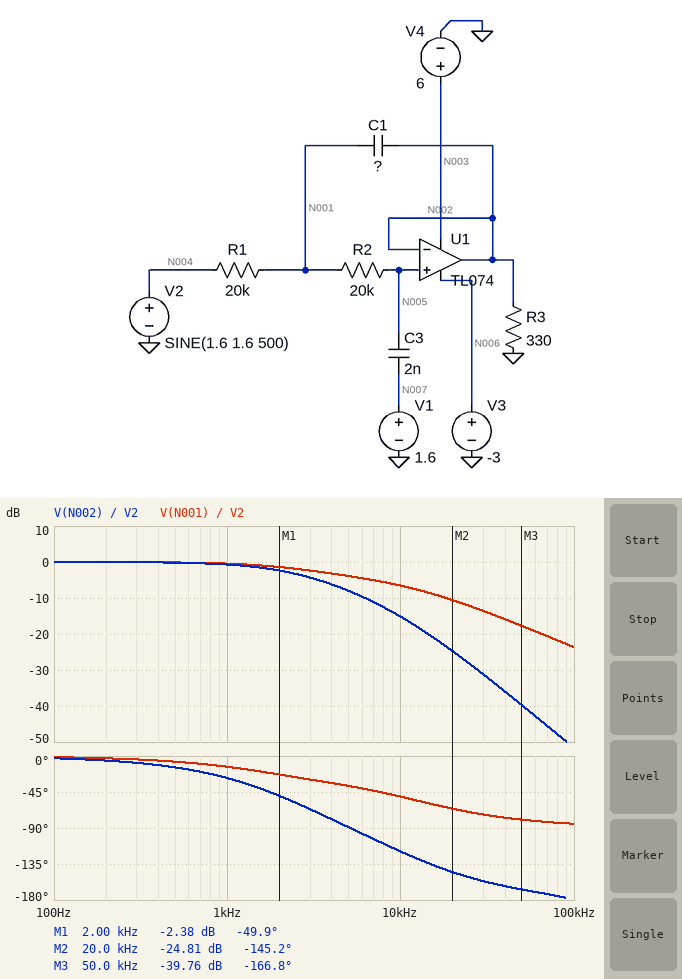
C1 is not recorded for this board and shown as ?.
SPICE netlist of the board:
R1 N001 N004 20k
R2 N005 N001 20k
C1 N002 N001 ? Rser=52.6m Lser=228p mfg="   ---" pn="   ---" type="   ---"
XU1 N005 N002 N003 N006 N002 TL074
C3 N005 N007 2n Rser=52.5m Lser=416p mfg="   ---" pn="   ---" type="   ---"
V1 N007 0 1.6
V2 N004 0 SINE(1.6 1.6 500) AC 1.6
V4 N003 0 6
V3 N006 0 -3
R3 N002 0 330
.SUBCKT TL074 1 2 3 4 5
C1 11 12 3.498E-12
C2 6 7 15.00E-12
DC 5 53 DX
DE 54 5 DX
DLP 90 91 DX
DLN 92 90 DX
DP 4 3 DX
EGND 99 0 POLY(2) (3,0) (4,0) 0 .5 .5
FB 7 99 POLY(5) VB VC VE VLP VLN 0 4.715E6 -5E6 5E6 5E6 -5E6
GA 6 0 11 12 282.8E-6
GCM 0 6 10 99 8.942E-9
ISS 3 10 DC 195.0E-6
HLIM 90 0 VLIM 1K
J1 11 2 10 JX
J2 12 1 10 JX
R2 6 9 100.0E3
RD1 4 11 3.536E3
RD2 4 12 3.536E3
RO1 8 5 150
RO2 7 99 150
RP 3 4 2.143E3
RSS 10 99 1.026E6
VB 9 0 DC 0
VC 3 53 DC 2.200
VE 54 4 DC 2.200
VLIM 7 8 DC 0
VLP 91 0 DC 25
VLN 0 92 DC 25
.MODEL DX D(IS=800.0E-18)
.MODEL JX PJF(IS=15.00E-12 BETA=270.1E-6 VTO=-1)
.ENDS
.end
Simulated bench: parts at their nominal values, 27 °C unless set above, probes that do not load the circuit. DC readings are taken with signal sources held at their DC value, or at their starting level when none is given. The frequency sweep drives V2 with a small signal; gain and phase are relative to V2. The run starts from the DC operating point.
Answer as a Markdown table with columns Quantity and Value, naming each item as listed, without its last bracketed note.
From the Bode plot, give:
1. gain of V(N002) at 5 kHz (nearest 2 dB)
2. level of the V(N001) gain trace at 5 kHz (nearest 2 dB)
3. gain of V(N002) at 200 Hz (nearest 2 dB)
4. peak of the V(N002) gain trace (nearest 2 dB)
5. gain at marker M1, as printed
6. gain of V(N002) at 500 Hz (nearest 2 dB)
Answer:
| Quantity | Value |
|---|---|
| gain of V(N002) at 5 kHz | -8 dB |
| level of the V(N001) gain trace at 5 kHz | -4 dB |
| gain of V(N002) at 200 Hz | 0 dB |
| peak of the V(N002) gain trace | 0 dB |
| gain at marker M1, as printed | -2.38 dB |
| gain of V(N002) at 500 Hz | 0 dB |
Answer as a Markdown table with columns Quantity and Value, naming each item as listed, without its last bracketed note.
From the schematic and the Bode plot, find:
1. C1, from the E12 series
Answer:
| Quantity | Value |
|---|---|
| C1, from the E12 series | 1.2 nF |
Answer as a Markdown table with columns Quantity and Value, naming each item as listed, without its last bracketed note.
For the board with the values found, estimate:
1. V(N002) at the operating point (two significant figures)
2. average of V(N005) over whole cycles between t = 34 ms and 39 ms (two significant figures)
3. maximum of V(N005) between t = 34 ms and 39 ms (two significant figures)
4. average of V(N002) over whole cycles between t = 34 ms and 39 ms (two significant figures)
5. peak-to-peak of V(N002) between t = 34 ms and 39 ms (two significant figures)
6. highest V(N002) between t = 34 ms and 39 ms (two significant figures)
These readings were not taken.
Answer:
| Quantity | Value |
|---|---|
| V(N002) at the operating point | 1.6 V |
| average of V(N005) over whole cycles between t = 34 ms and 39 ms | 1.6 V |
| maximum of V(N005) between t = 34 ms and 39 ms | 3.2 V |
| average of V(N002) over whole cycles between t = 34 ms and 39 ms | 1.6 V |
| peak-to-peak of V(N002) between t = 34 ms and 39 ms | 3.1 V |
| highest V(N002) between t = 34 ms and 39 ms | 3.2 V |
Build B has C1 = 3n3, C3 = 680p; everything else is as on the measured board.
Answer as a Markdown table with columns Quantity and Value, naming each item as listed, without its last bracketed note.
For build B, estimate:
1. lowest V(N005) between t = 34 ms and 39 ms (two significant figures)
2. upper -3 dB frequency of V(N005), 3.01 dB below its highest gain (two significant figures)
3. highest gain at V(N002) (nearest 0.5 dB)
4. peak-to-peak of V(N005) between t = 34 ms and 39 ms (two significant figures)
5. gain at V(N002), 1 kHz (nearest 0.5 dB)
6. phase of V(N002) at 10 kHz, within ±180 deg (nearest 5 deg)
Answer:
| Quantity | Value |
|---|---|
| lowest V(N005) between t = 34 ms and 39 ms | -8.4 mV |
| upper -3 dB frequency of V(N005), 3.01 dB below its highest gain | 6.3 kHz |
| highest gain at V(N002) | 2.0 dB |
| peak-to-peak of V(N005) between t = 34 ms and 39 ms | 3.2 V |
| gain at V(N002), 1 kHz | 0 dB |
| phase of V(N002) at 10 kHz, within ±180 deg | -145 deg |
